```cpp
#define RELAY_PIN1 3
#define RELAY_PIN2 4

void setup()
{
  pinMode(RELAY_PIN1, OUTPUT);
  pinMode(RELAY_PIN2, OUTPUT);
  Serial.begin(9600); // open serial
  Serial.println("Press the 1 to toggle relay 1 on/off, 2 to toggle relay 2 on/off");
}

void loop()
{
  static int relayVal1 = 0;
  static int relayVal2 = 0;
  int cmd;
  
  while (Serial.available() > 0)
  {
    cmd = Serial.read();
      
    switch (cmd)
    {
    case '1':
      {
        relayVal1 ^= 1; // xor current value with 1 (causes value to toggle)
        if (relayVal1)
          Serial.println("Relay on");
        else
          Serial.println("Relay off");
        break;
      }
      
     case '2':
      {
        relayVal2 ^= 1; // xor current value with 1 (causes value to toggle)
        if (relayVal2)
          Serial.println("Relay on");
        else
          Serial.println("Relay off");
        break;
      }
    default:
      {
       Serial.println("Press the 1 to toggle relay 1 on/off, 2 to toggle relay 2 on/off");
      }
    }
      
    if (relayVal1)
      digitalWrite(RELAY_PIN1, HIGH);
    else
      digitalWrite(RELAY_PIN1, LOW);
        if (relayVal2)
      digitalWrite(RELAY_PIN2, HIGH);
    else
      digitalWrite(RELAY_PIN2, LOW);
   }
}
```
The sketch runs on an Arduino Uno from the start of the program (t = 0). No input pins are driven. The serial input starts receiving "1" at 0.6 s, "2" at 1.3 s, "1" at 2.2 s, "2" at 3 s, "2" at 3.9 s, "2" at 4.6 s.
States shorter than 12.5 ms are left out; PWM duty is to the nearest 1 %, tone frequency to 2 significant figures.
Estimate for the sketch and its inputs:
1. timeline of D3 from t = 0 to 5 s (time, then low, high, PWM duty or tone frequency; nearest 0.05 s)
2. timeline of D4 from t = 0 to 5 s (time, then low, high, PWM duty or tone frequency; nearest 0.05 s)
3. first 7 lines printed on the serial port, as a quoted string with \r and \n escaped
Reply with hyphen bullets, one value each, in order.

- 0 s low; 0.6 s high; 2.2 s low
- 0 s low; 1.3 s high; 3 s low; 3.9 s high; 4.6 s low
- "Press the 1 to toggle relay 1 on/off, 2 to toggle relay 2 on/off\r\nRelay on\r\nRelay on\r\nRelay off\r\nRelay off\r\nRelay on\r\nRelay off\r\n"
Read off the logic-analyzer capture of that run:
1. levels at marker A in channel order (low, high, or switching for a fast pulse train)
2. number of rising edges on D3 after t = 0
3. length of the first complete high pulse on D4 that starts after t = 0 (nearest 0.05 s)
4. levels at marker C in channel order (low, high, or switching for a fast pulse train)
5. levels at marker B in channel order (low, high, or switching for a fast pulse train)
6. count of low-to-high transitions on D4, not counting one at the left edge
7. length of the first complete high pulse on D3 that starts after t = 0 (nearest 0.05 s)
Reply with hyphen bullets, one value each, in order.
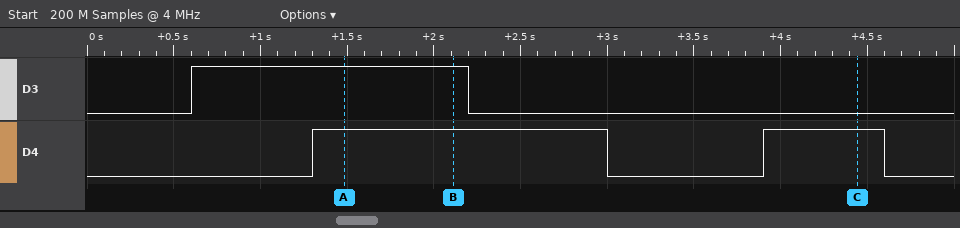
- D3 high, D4 high
- 1
- 1.70 s
- D3 low, D4 high
- D3 high, D4 high
- 2
- 1.60 s
